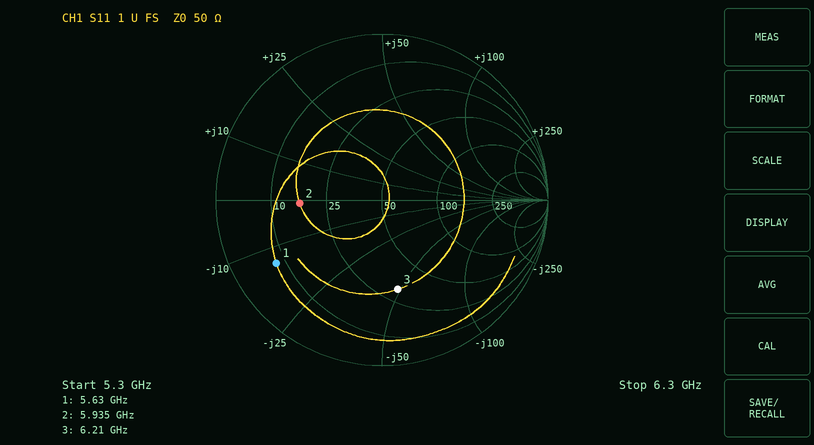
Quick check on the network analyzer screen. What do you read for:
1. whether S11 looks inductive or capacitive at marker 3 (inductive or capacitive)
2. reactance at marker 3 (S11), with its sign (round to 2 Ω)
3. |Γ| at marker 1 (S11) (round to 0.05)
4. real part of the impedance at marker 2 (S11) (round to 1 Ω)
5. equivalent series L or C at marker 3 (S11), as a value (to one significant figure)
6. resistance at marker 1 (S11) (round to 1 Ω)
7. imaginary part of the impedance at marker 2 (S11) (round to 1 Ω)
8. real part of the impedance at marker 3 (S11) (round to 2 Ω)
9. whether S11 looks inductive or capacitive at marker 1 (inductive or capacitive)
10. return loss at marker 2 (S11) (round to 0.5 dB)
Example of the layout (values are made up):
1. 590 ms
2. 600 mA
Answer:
1. capacitive
2. -48 Ω
3. 0.75
4. 17 Ω
5. 500 fF
6. 8 Ω
7. -1 Ω
8. 32 Ω
9. capacitive
10. 6.0 dB
